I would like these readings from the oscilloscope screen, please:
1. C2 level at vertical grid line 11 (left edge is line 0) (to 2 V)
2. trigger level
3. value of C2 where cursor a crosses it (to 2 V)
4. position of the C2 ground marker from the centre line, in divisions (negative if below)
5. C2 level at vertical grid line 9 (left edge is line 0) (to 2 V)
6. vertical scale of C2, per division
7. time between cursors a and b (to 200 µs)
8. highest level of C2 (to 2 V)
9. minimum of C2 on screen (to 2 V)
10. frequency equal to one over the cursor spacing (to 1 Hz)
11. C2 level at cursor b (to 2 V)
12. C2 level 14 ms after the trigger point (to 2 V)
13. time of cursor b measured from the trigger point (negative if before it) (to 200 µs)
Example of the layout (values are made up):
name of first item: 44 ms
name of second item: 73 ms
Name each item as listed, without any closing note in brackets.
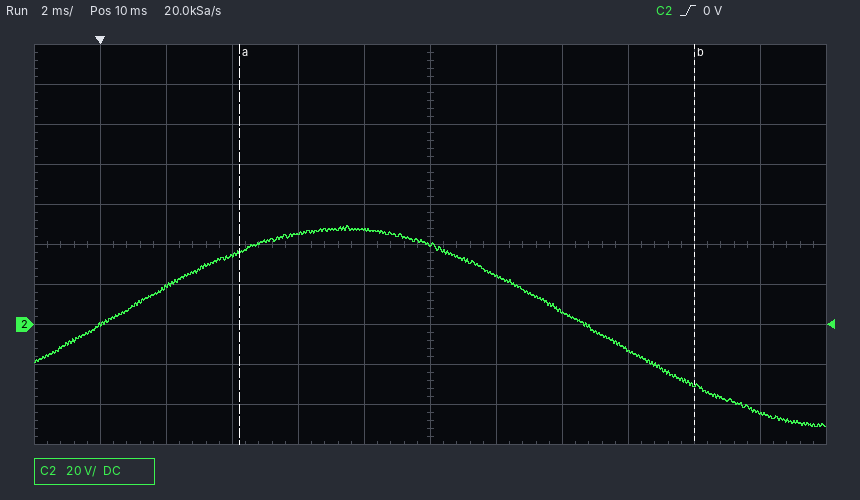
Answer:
C2 level at vertical grid line 11 (left edge is line 0): -44 V
trigger level: 0 V
value of C2 where cursor a crosses it: 36 V
position of the C2 ground marker from the centre line, in divisions: -2.0 div
C2 level at vertical grid line 9 (left edge is line 0): -12 V
vertical scale of C2, per division: 20 V
time between cursors a and b: 13.8 ms
highest level of C2: 50 V
minimum of C2 on screen: -52 V
frequency equal to one over the cursor spacing: 72 Hz
C2 level at cursor b: -30 V
C2 level 14 ms after the trigger point: 6 V
time of cursor b measured from the trigger point (negative if before it): +18.0 ms
